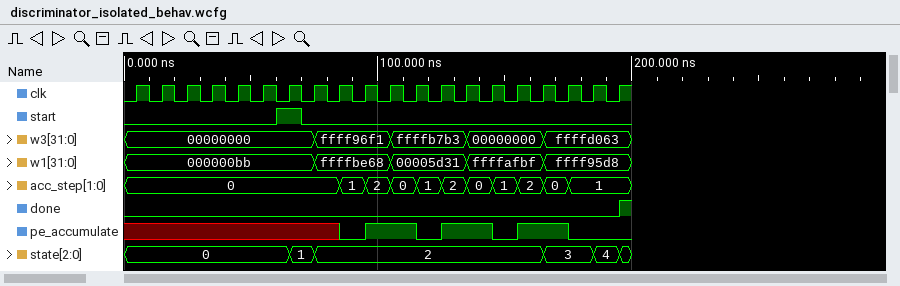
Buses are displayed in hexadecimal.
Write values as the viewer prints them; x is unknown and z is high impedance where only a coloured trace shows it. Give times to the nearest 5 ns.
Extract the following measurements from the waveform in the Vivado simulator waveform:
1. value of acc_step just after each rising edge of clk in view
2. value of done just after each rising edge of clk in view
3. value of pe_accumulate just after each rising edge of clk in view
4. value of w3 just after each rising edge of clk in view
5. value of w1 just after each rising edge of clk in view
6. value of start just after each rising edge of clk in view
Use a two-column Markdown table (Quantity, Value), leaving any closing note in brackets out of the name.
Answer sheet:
| Quantity | Value |
|---|---|
| value of acc_step just after each rising edge of clk in view | 0, 0, 0, 0, 0, 0, 0, 0, 1, 2, 0, 1, 2, 0, 1, 2, 0, 1, 1, 1 |
| value of done just after each rising edge of clk in view | 0 0 0 0 0 0 0 0 0 0 0 0 0 0 0 0 0 0 0 1 |
| value of pe_accumulate just after each rising edge of clk in view | x x x x x x x x 0 1 1 0 1 1 0 1 1 0 0 0 |
| value of w3 just after each rising edge of clk in view | 00000000, 00000000, 00000000, 00000000, 00000000, 00000000, 00000000, ffff96f1, ffff96f1, ffff96f1, ffffb7b3, ffffb7b3, ffffb7b3, 00000000, 00000000, 00000000, ffffd063, ffffd063, ffffd063, ffffd063 |
| value of w1 just after each rising edge of clk in view | 000000bb, 000000bb, 000000bb, 000000bb, 000000bb, 000000bb, 000000bb, ffffbe68, ffffbe68, ffffbe68, 00005d31, 00005d31, 00005d31, ffffafbf, ffffafbf, ffffafbf, ffff95d8, ffff95d8, ffff95d8, ffff95d8 |
| value of start just after each rising edge of clk in view | 0 0 0 0 0 0 1 0 0 0 0 0 0 0 0 0 0 0 0 0 |
